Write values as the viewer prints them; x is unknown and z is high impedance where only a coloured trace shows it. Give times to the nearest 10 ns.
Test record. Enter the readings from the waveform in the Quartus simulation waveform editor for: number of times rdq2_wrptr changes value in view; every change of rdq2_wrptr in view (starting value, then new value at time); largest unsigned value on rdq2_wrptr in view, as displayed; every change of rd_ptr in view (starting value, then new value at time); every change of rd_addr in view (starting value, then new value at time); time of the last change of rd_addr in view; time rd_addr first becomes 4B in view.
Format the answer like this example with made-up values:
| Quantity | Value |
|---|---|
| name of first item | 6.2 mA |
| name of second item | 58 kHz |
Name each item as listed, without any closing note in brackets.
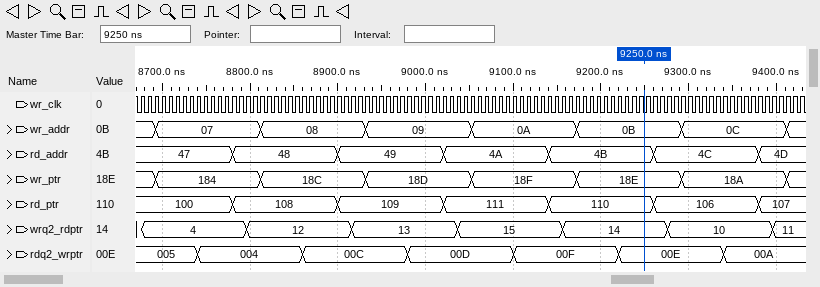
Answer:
| Quantity | Value |
|---|---|
| number of times rdq2_wrptr changes value in view | 6 |
| every change of rdq2_wrptr in view | 005, 004 at 8740 ns, 00C at 8860 ns, 00D at 8980 ns, 00F at 9100 ns, 00E at 9220 ns, 00A at 9340 ns |
| largest unsigned value on rdq2_wrptr in view, as displayed | 00F |
| every change of rd_ptr in view | 100, 108 at 8780 ns, 109 at 8900 ns, 111 at 9020 ns, 110 at 9140 ns, 106 at 9260 ns, 107 at 9380 ns |
| every change of rd_addr in view | 47, 48 at 8780 ns, 49 at 8900 ns, 4A at 9020 ns, 4B at 9140 ns, 4C at 9260 ns, 4D at 9380 ns |
| time of the last change of rd_addr in view | 9380 ns |
| time rd_addr first becomes 4B in view | 9140 ns |
